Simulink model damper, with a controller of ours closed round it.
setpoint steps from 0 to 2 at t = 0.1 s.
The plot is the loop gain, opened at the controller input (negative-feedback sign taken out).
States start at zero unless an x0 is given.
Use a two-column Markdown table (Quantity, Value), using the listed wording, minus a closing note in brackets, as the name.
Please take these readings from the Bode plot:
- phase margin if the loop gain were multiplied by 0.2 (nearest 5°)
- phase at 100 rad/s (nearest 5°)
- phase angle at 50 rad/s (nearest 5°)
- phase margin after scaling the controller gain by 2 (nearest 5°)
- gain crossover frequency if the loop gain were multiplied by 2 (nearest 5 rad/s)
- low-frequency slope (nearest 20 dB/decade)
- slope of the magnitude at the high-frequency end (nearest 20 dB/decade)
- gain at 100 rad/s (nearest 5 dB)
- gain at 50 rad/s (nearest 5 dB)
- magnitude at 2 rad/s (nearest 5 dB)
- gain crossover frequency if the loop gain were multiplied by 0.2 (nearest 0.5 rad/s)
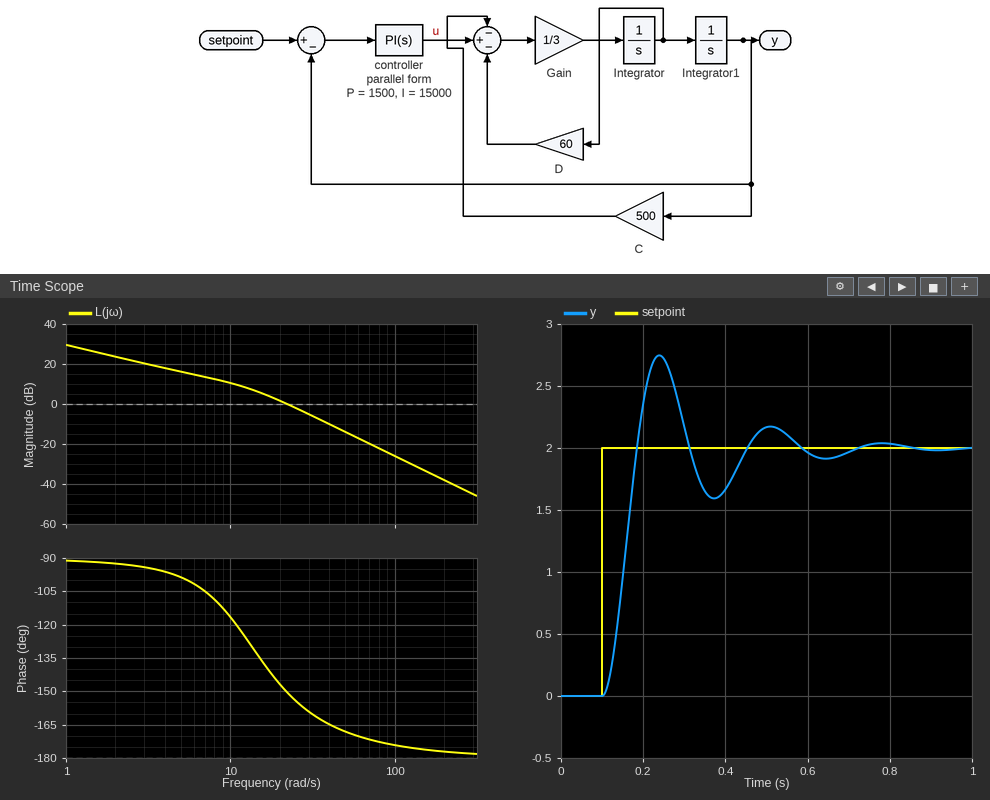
| Quantity | Value |
|---|---|
| phase margin if the loop gain were multiplied by 0.2 | 75° |
| phase at 100 rad/s | -175° |
| phase angle at 50 rad/s | -170° |
| phase margin after scaling the controller gain by 2 | 20° |
| gain crossover frequency if the loop gain were multiplied by 2 | 30 rad/s |
| low-frequency slope | -20 dB/decade |
| slope of the magnitude at the high-frequency end | -40 dB/decade |
| gain at 100 rad/s | -25 dB |
| gain at 50 rad/s | -15 dB |
| magnitude at 2 rad/s | 25 dB |
| gain crossover frequency if the loop gain were multiplied by 0.2 | 6.5 rad/s |
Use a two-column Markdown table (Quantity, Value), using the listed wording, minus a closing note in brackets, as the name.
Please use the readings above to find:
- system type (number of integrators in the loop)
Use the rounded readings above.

| Quantity | Value |
|---|---|
| system type | 1 |
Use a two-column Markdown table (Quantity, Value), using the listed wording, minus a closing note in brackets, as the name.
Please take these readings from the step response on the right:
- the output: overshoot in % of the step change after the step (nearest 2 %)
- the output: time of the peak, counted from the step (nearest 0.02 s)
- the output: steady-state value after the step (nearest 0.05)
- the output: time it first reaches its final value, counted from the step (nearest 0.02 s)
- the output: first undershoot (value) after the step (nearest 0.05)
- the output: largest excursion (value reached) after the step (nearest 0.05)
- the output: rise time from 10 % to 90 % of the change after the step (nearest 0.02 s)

| Quantity | Value |
|---|---|
| the output: overshoot in % of the step change after the step | 38 % |
| the output: time of the peak, counted from the step | 0.14 s |
| the output: steady-state value after the step | 2.00 |
| the output: time it first reaches its final value, counted from the step | 0.08 s |
| the output: first undershoot (value) after the step | 1.60 |
| the output: largest excursion (value reached) after the step | 2.75 |
| the output: rise time from 10 % to 90 % of the change after the step | 0.06 s |
